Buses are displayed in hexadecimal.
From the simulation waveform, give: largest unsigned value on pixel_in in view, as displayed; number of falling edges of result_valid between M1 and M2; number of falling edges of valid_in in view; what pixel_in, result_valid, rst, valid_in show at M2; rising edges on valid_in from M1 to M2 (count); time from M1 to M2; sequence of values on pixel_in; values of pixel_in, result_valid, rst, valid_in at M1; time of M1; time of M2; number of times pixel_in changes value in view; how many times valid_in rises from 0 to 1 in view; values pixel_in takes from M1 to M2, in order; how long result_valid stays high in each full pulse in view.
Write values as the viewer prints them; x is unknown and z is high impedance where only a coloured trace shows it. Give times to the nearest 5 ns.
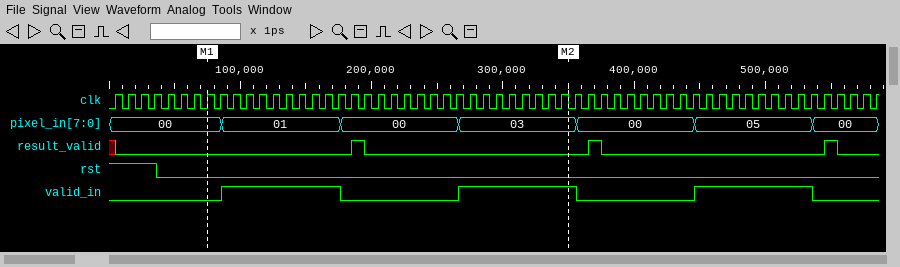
05
1
3
pixel_in=03, result_valid=0, rst=0, valid_in=1
2
275 ns
00, 01, 00, 03, 00, 05, 00
pixel_in=00, result_valid=0, rst=0, valid_in=0
75 ns
350 ns
6
3
00, 01, 00, 03
10 ns, 10 ns, 10 ns
